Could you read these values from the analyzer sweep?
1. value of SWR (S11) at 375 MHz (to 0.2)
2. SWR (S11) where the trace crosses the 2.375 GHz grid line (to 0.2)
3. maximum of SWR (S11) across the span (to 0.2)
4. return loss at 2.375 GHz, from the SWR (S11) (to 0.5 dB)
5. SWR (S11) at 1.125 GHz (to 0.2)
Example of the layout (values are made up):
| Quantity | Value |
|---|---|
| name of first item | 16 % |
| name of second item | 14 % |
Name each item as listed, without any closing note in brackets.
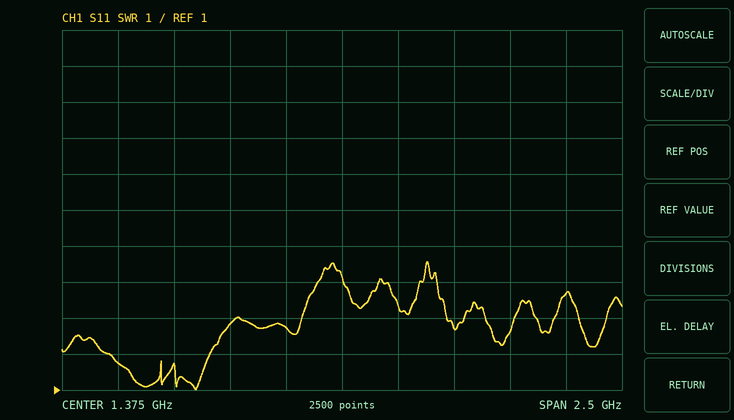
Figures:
| Quantity | Value |
|---|---|
| value of SWR (S11) at 375 MHz | 1.8 |
| SWR (S11) where the trace crosses the 2.375 GHz grid line | 3.6 |
| maximum of SWR (S11) across the span | 4.6 |
| return loss at 2.375 GHz, from the SWR (S11) | 5.0 dB |
| SWR (S11) at 1.125 GHz | 2.8 |
